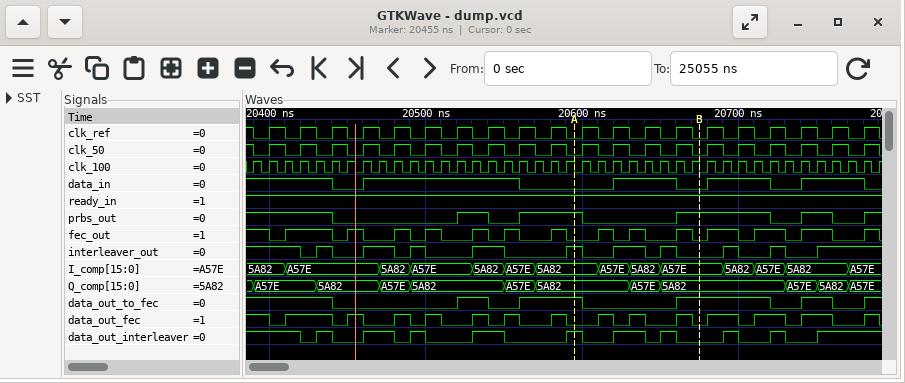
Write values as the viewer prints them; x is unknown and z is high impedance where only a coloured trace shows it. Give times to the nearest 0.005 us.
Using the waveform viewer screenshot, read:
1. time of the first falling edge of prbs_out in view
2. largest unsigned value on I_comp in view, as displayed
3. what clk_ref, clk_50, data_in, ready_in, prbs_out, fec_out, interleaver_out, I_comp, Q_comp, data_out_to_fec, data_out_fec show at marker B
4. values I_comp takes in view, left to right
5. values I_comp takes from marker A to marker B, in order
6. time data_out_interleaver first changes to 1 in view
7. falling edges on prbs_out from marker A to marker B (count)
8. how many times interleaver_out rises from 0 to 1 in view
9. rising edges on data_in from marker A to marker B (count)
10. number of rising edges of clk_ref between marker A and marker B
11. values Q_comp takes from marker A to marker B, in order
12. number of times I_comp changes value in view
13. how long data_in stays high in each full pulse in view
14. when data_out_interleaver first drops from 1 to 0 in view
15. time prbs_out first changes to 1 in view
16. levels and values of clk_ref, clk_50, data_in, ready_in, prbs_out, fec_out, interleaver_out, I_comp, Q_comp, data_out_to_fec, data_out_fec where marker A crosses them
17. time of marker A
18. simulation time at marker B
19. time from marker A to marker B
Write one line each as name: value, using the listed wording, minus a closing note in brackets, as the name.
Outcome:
time of the first falling edge of prbs_out in view: 20.44 us
largest unsigned value on I_comp in view, as displayed: A57E
what clk_ref, clk_50, data_in, ready_in, prbs_out, fec_out, interleaver_out, I_comp, Q_comp, data_out_to_fec, data_out_fec show at marker B: clk_ref=0, clk_50=0, data_in=0, ready_in=1, prbs_out=1, fec_out=0, interleaver_out=0, I_comp=A57E, Q_comp=5A82, data_out_to_fec=1, data_out_fec=0
values I_comp takes in view, left to right: 5A82, A57E, 5A82, A57E, 5A82, A57E, 5A82, A57E, 5A82, A57E, 5A82, A57E, 5A82, A57E
values I_comp takes from marker A to marker B, in order: 5A82, A57E, 5A82, A57E
time data_out_interleaver first changes to 1 in view: 20.43 us
falling edges on prbs_out from marker A to marker B: 1
how many times interleaver_out rises from 0 to 1 in view: 10
rising edges on data_in from marker A to marker B: 1
number of rising edges of clk_ref between marker A and marker B: 4
values Q_comp takes from marker A to marker B, in order: 5A82, A57E, 5A82
number of times I_comp changes value in view: 13
how long data_in stays high in each full pulse in view: 0.1 us, 0.04 us, 0.04 us, 0.04 us
when data_out_interleaver first drops from 1 to 0 in view: 20.42 us
time prbs_out first changes to 1 in view: 20.52 us
levels and values of clk_ref, clk_50, data_in, ready_in, prbs_out, fec_out, interleaver_out, I_comp, Q_comp, data_out_to_fec, data_out_fec where marker A crosses them: clk_ref=0, clk_50=0, data_in=0, ready_in=1, prbs_out=1, fec_out=0, interleaver_out=1, I_comp=5A82, Q_comp=5A82, data_out_to_fec=1, data_out_fec=0
time of marker A: 20.595 us
simulation time at marker B: 20.675 us
time from marker A to marker B: 0.08 us
